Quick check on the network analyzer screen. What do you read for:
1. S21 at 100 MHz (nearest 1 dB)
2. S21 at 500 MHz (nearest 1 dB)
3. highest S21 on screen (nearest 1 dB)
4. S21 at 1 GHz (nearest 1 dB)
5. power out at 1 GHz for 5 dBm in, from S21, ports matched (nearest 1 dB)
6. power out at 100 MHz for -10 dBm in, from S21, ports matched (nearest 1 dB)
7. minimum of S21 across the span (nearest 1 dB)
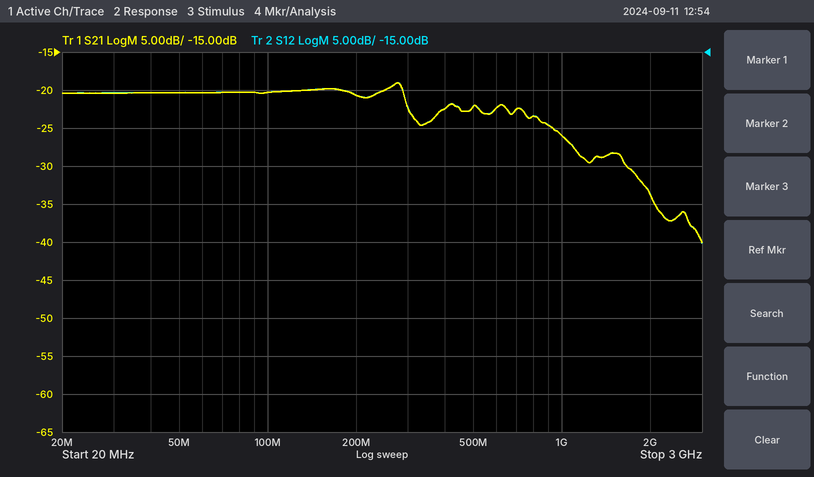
-20 dB
-22 dB
-19 dB
-26 dB
-21 dBm
-30 dBm
-40 dB
